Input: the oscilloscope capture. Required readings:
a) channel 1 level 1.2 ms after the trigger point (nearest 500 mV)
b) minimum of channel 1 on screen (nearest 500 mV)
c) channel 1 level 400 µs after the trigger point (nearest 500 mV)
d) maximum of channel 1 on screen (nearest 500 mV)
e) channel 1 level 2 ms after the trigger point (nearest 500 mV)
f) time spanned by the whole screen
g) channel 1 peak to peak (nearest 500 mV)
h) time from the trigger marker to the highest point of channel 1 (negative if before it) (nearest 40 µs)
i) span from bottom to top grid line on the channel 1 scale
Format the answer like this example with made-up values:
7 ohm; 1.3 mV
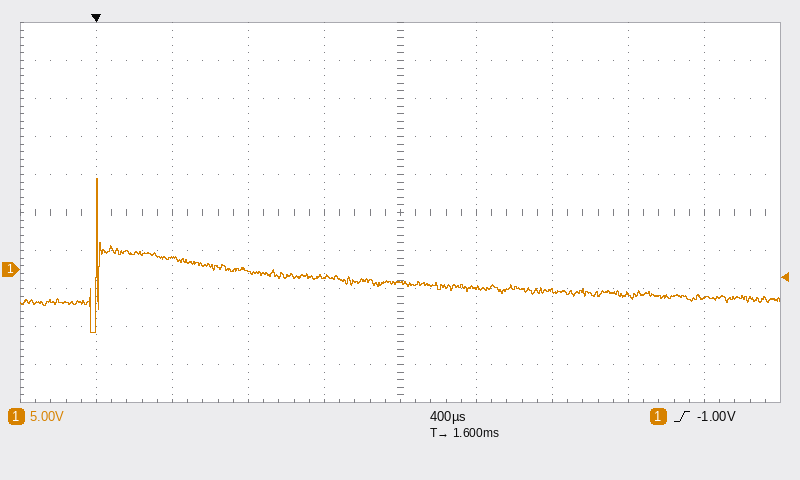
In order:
-1.0 V; -8.5 V; 1.5 V; 12.0 V; -2.5 V; 4 ms; 20.5 V; 0 µs; 50 V
